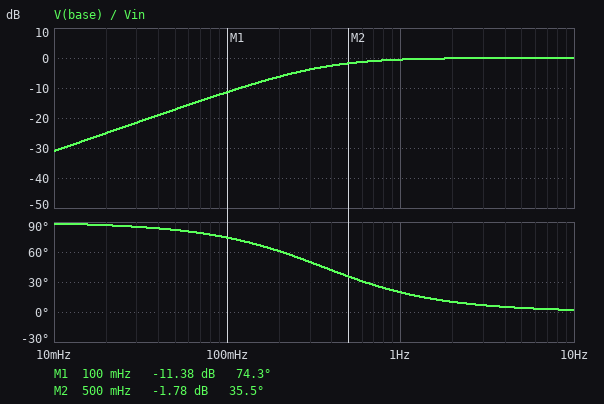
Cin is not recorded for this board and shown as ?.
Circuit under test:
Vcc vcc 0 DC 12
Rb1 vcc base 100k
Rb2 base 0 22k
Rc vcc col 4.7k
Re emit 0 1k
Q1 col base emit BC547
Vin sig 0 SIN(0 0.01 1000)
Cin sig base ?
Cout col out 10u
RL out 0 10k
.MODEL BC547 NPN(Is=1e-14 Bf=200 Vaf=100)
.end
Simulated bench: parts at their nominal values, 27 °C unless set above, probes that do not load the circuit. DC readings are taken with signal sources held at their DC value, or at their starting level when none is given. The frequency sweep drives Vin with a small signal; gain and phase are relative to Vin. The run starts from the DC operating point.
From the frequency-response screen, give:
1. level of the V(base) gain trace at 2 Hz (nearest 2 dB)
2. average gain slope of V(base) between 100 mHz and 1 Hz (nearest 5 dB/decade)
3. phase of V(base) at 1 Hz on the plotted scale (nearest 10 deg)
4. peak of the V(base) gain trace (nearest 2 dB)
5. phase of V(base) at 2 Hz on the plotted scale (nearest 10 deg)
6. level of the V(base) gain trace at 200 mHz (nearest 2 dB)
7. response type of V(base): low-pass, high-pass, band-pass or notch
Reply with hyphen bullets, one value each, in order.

- 0 dB
- 10 dB/decade
- 20 deg
- 0 dB
- 10 deg
- -6 dB
- high-pass
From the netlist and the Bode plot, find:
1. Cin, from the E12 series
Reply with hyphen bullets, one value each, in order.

- 27 µF
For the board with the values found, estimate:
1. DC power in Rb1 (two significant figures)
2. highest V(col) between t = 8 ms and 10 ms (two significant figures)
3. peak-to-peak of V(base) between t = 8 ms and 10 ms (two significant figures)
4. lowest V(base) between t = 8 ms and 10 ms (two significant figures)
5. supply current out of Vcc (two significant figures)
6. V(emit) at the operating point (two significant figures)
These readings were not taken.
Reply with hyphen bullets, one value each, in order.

- 990 µW
- 5.6 V
- 20 mV
- 2.0 V
- 1.5 mA
- 1.4 V
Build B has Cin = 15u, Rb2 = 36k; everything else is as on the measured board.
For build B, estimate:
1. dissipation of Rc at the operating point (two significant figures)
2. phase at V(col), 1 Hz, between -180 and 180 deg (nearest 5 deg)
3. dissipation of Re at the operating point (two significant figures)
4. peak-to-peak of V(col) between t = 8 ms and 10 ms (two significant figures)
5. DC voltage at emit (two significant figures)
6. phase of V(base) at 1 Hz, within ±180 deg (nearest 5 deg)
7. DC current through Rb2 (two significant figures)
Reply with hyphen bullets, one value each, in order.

- 20 mW
- -100 deg
- 4.4 mW
- 32 mV
- 2.1 V
- 85 deg
- 77 µA
